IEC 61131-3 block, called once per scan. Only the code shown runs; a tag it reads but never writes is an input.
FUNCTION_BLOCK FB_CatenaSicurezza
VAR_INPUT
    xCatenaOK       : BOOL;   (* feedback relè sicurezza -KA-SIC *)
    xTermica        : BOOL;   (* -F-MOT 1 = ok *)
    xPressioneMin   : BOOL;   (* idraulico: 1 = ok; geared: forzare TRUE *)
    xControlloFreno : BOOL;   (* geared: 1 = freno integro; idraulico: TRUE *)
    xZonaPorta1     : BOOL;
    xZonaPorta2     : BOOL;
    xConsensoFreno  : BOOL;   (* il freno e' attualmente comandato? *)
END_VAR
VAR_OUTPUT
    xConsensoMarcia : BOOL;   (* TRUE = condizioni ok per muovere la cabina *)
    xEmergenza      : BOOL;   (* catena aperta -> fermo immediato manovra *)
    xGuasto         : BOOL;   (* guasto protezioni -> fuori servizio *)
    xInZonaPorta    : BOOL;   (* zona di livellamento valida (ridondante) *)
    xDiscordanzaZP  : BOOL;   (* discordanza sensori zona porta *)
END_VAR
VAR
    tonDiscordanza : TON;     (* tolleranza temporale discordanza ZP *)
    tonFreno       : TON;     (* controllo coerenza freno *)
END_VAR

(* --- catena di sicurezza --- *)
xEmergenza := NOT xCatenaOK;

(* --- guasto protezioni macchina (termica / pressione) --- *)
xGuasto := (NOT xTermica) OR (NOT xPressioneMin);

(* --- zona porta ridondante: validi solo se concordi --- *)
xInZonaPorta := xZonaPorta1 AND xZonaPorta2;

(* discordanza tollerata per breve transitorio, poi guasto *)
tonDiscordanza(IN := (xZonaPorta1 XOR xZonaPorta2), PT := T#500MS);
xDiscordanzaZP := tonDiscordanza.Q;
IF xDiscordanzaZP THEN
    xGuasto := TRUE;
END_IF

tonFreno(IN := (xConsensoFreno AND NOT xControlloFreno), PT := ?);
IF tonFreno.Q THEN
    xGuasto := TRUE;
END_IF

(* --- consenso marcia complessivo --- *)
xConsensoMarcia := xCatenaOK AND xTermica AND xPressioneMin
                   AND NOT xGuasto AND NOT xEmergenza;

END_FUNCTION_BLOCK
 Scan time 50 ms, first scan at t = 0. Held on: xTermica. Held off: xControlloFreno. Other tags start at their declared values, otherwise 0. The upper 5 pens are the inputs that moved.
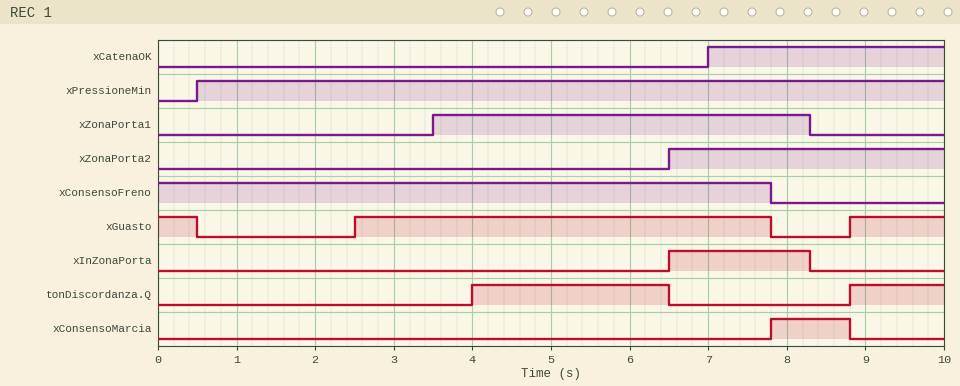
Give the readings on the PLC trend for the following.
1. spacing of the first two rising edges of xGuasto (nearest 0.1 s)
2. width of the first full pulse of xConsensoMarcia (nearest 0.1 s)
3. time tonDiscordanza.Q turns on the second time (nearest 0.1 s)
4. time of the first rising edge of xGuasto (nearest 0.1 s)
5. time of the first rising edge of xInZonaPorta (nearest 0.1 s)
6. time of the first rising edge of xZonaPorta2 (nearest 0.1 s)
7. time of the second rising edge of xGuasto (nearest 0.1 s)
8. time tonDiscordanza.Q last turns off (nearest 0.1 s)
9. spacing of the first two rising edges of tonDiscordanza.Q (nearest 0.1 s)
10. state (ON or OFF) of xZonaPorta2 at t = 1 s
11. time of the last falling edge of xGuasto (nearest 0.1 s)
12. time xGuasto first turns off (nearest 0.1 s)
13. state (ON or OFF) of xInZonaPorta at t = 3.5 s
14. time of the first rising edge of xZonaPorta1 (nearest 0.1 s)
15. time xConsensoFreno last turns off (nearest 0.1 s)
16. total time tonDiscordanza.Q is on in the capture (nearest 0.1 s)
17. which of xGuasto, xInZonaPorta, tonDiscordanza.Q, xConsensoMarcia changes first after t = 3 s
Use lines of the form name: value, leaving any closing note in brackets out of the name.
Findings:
spacing of the first two rising edges of xGuasto: 6.3 s
width of the first full pulse of xConsensoMarcia: 1.0 s
time tonDiscordanza.Q turns on the second time: 8.8 s
time of the first rising edge of xGuasto: 2.5 s
time of the first rising edge of xInZonaPorta: 6.5 s
time of the first rising edge of xZonaPorta2: 6.5 s
time of the second rising edge of xGuasto: 8.8 s
time tonDiscordanza.Q last turns off: 6.5 s
spacing of the first two rising edges of tonDiscordanza.Q: 4.8 s
state (ON or OFF) of xZonaPorta2 at t = 1 s: OFF
time of the last falling edge of xGuasto: 7.8 s
time xGuasto first turns off: 0.5 s
state (ON or OFF) of xInZonaPorta at t = 3.5 s: OFF
time of the first rising edge of xZonaPorta1: 3.5 s
time xConsensoFreno last turns off: 7.8 s
total time tonDiscordanza.Q is on in the capture: 3.7 s
which of xGuasto, xInZonaPorta, tonDiscordanza.Q, xConsensoMarcia changes first after t = 3 s: tonDiscordanza.Q
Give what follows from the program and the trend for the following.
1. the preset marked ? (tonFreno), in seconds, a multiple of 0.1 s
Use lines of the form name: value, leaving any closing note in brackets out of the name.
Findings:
the preset marked ? (tonFreno), in seconds, a multiple of 0.1 s: 2.5 s
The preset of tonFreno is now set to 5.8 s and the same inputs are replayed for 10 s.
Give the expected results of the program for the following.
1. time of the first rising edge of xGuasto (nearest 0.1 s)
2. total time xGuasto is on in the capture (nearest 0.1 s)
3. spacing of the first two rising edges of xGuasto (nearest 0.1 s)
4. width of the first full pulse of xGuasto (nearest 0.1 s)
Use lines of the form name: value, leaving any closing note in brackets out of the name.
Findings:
time of the first rising edge of xGuasto: 4.0 s
total time xGuasto is on in the capture: 5.5 s
spacing of the first two rising edges of xGuasto: 4.8 s
width of the first full pulse of xGuasto: 3.8 s
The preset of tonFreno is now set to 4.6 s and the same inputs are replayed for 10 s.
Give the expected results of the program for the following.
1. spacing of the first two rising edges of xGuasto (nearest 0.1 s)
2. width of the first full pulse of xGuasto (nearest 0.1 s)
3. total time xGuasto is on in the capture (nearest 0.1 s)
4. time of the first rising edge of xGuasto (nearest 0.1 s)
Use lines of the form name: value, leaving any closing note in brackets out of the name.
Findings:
spacing of the first two rising edges of xGuasto: 4.8 s
width of the first full pulse of xGuasto: 3.8 s
total time xGuasto is on in the capture: 5.5 s
time of the first rising edge of xGuasto: 4.0 s
